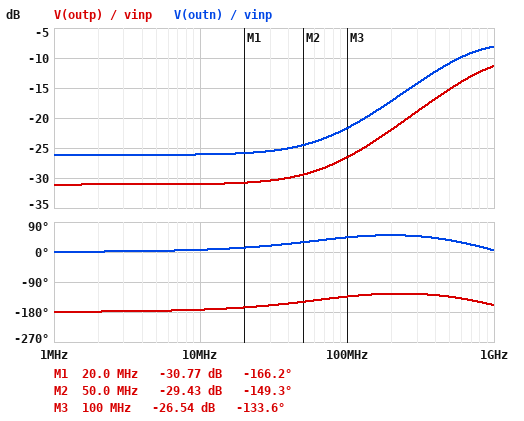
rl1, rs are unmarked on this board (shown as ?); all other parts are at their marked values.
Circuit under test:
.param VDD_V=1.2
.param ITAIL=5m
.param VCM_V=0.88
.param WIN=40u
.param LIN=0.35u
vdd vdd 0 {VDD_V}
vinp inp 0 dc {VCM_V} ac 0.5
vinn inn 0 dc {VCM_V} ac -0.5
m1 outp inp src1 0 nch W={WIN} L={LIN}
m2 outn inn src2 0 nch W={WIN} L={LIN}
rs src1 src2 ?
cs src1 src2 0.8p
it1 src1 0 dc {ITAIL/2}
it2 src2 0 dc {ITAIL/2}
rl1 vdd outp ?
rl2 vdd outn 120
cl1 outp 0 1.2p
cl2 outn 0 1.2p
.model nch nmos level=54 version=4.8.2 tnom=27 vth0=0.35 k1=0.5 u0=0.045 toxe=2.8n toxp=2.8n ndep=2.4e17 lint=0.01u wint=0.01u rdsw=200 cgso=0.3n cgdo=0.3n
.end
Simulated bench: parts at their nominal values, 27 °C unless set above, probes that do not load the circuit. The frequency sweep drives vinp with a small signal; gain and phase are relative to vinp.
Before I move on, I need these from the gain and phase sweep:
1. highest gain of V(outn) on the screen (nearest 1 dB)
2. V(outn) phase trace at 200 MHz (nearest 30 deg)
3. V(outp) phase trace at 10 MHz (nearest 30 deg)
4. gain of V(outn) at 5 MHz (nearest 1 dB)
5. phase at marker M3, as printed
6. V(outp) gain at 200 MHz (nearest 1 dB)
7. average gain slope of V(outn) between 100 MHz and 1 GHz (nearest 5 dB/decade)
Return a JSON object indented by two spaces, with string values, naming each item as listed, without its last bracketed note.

{
  "highest gain of V(outn) on the screen": "-8 dB",
  "V(outn) phase trace at 200 MHz": "60 deg",
  "V(outp) phase trace at 10 MHz": "-180 deg",
  "gain of V(outn) at 5 MHz": "-26 dB",
  "phase at marker M3, as printed": "-133.6 deg",
  "V(outp) gain at 200 MHz": "-22 dB",
  "average gain slope of V(outn) between 100 MHz and 1 GHz": "15 dB/decade"
}
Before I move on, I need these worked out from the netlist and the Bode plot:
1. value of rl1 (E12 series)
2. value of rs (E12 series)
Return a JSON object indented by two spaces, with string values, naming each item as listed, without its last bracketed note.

{
  "value of rl1": "68 Ω",
  "value of rs": "2.7 kΩ"
}
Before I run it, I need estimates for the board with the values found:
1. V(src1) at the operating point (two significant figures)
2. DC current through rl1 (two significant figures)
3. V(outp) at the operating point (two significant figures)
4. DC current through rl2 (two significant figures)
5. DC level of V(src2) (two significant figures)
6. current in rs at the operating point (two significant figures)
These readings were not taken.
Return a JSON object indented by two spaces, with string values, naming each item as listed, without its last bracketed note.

{
  "V(src1) at the operating point": "56 mV",
  "DC current through rl1": "2.5 mA",
  "V(outp) at the operating point": "1.0 V",
  "DC current through rl2": "2.5 mA",
  "DC level of V(src2)": "53 mV",
  "current in rs at the operating point": "1.3 µA"
}
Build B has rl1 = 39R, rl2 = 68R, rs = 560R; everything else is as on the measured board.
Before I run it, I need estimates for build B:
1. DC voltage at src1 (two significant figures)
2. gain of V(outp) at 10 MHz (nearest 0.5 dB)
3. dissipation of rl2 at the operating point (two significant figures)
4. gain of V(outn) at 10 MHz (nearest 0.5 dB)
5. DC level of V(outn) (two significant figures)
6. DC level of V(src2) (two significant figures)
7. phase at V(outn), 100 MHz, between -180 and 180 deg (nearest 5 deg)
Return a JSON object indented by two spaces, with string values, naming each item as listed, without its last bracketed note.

{
  "DC voltage at src1": "58 mV",
  "gain of V(outp) at 10 MHz": "-23.5 dB",
  "dissipation of rl2 at the operating point": "420 µW",
  "gain of V(outn) at 10 MHz": "-19.0 dB",
  "DC level of V(outn)": "1.0 V",
  "DC level of V(src2)": "56 mV",
  "phase at V(outn), 100 MHz, between -180 and 180 deg": "10 deg"
}
